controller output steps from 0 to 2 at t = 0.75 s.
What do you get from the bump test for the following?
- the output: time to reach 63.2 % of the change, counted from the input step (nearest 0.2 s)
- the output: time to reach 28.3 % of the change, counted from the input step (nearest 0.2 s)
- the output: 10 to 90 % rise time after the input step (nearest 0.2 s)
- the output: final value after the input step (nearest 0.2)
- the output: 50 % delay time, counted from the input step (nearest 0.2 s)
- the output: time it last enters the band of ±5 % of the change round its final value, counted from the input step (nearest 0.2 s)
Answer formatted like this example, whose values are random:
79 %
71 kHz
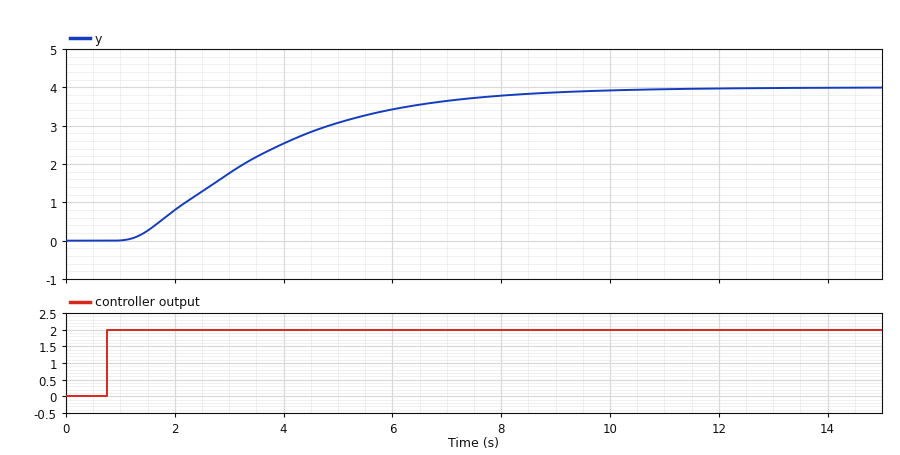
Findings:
3.2 s
1.6 s
5.2 s
4.0
2.6 s
7.4 s
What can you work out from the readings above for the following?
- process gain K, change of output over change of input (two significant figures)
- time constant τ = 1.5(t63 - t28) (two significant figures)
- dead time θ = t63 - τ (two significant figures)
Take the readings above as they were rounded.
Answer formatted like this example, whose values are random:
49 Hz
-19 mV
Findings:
2.0
2.4 s
0.80 s
